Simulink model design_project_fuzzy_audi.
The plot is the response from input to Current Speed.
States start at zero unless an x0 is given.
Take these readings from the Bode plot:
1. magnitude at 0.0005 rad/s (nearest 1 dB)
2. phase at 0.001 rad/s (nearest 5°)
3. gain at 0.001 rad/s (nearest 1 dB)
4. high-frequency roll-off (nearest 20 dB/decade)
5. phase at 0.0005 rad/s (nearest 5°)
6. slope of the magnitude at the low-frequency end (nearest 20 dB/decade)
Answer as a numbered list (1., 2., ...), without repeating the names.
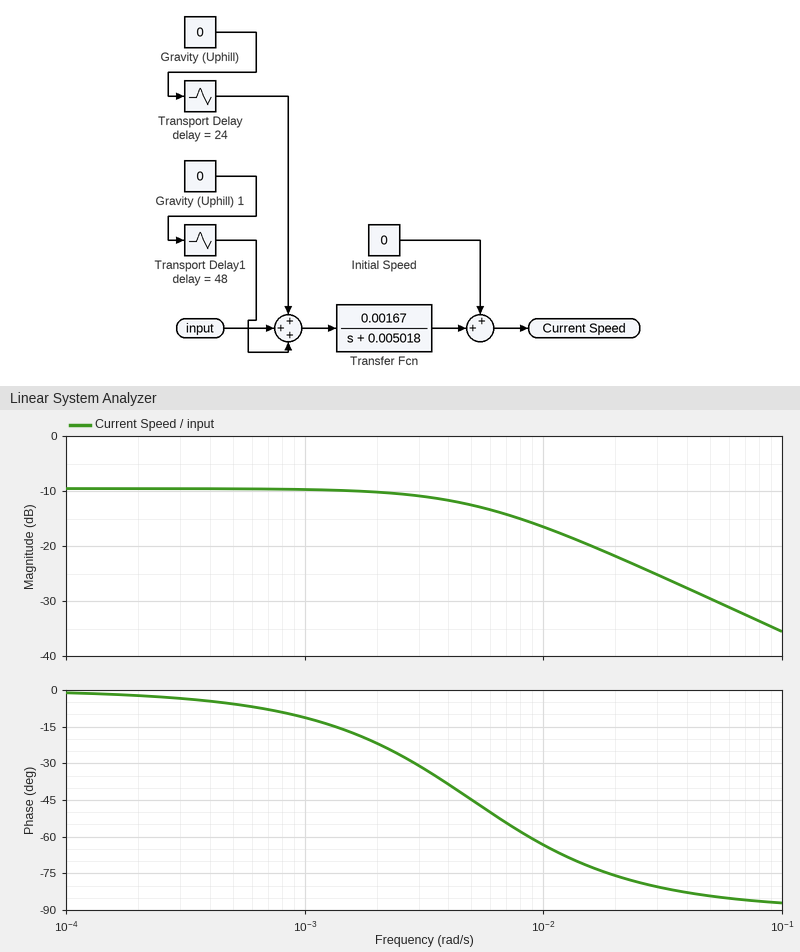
1. -10 dB
2. -10°
3. -10 dB
4. -20 dB/decade
5. -5°
6. 0 dB/decade
